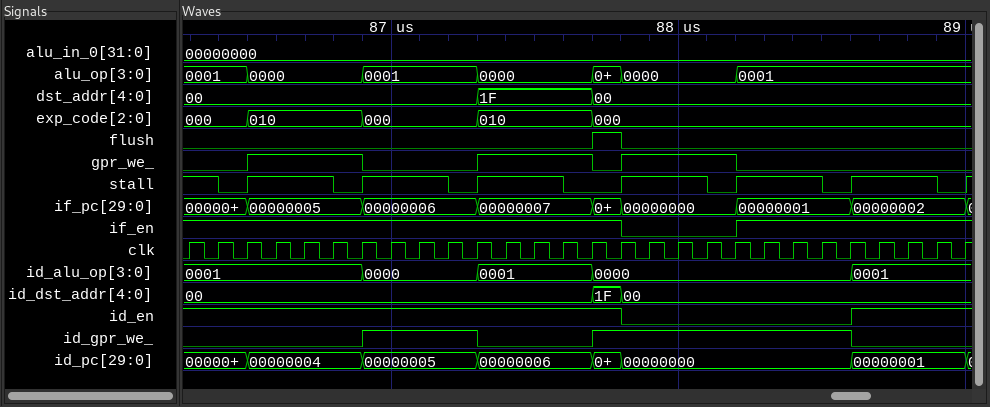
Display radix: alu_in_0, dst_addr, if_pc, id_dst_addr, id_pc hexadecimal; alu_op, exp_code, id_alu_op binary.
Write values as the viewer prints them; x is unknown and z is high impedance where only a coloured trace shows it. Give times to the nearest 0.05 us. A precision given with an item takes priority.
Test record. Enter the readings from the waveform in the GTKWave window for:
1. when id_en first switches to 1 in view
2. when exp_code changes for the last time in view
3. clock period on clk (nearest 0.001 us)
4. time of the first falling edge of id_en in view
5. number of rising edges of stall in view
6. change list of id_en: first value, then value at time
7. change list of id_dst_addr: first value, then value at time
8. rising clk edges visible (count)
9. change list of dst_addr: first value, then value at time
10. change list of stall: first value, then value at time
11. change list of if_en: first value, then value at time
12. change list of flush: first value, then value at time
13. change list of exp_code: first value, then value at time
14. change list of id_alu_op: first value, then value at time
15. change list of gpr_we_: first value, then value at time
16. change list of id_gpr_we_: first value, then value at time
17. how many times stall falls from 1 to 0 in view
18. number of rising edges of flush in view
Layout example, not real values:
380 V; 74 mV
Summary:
88.6 us; 87.7 us; 0.1 us; 87.8 us; 7; 1, 0 at 87.8 us, 1 at 88.6 us; 00, 1F at 87.7 us, 00 at 87.8 us; 28; 00, 1F at 87.3 us, 00 at 87.7 us; 1, 0 at 86.4 us, 1 at 86.5 us, 0 at 86.8 us, 1 at 86.9 us, 0 at 87.2 us, 1 at 87.3 us, 0 at 87.6 us, 1 at 87.8 us, 0 at 88.1 us, 1 at 88.2 us, 0 at 88.5 us, 1 at 88.6 us, 0 at 88.9 us, 1 at 89 us; 1, 0 at 87.8 us, 1 at 88.2 us; 0, 1 at 87.7 us, 0 at 87.8 us; 000, 010 at 86.5 us, 000 at 86.9 us, 010 at 87.3 us, 000 at 87.7 us; 0001, 0000 at 86.9 us, 0001 at 87.3 us, 0000 at 87.7 us, 0001 at 88.6 us; 0, 1 at 86.5 us, 0 at 86.9 us, 1 at 87.3 us, 0 at 87.7 us, 1 at 87.8 us, 0 at 88.2 us; 0, 1 at 86.9 us, 0 at 87.3 us, 1 at 87.7 us, 0 at 88.6 us; 7; 1
